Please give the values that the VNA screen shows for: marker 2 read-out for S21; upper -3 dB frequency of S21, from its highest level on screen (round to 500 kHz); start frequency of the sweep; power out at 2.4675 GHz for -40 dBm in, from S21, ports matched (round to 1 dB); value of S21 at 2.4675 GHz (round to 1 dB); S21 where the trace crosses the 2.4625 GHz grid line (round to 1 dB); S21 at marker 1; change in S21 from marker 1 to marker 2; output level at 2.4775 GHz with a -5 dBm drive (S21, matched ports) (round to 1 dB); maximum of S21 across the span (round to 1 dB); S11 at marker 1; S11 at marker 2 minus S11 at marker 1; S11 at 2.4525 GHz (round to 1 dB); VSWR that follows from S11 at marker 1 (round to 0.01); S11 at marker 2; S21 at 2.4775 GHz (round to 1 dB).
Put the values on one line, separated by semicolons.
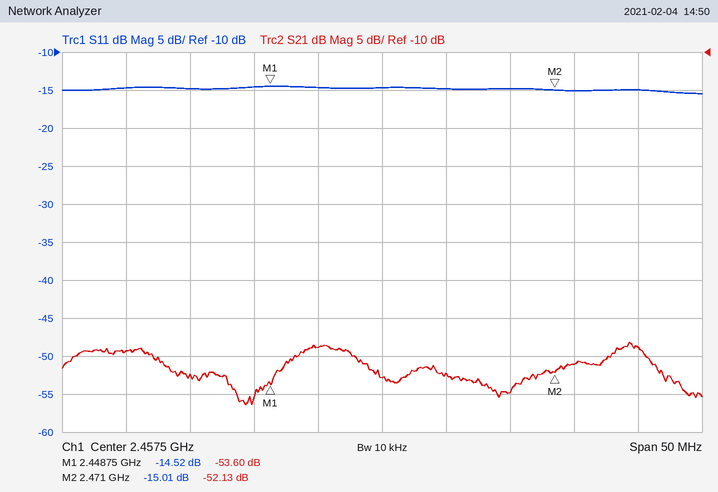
-52.13 dB; 2.4790 GHz; 2.4325 GHz; -95 dBm; -55 dB; -52 dB; -53.60 dB; 1.47 dB; -54 dBm; -48 dB; -14.52 dB; -0.49 dB; -15 dB; 1.46; -15.01 dB; -49 dB
